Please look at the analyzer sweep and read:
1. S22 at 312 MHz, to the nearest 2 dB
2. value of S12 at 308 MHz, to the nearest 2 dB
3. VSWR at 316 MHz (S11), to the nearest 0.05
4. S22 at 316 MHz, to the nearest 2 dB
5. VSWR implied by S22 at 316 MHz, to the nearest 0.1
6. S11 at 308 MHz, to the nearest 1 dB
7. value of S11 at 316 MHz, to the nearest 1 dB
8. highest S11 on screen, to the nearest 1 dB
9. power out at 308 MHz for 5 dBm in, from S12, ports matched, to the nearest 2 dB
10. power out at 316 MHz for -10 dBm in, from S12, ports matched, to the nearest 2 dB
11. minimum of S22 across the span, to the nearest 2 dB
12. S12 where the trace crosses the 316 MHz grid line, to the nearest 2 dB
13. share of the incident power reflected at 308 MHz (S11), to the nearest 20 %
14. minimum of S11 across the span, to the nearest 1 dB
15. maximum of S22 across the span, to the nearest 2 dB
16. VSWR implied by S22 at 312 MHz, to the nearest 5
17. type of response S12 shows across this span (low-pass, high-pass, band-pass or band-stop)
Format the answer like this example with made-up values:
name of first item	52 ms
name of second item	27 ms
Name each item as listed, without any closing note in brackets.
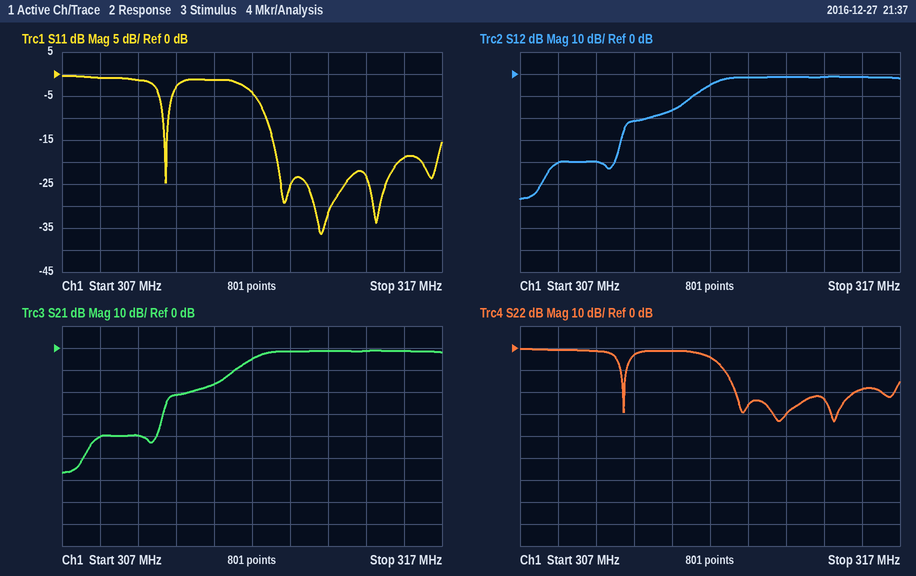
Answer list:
S22 at 312 MHz, to the nearest 2 dB	-4 dB
value of S12 at 308 MHz, to the nearest 2 dB	-40 dB
VSWR at 316 MHz (S11), to the nearest 0.05	1.25
S22 at 316 MHz, to the nearest 2 dB	-18 dB
VSWR implied by S22 at 316 MHz, to the nearest 0.1	1.3
S11 at 308 MHz, to the nearest 1 dB	-1 dB
value of S11 at 316 MHz, to the nearest 1 dB	-19 dB
highest S11 on screen, to the nearest 1 dB	0 dB
power out at 308 MHz for 5 dBm in, from S12, ports matched, to the nearest 2 dB	-36 dBm
power out at 316 MHz for -10 dBm in, from S12, ports matched, to the nearest 2 dB	-12 dBm
minimum of S22 across the span, to the nearest 2 dB	-34 dB
S12 where the trace crosses the 316 MHz grid line, to the nearest 2 dB	-2 dB
share of the incident power reflected at 308 MHz (S11), to the nearest 20 %	80 %
minimum of S11 across the span, to the nearest 1 dB	-36 dB
maximum of S22 across the span, to the nearest 2 dB	0 dB
VSWR implied by S22 at 312 MHz, to the nearest 5	5
type of response S12 shows across this span	high-pass
